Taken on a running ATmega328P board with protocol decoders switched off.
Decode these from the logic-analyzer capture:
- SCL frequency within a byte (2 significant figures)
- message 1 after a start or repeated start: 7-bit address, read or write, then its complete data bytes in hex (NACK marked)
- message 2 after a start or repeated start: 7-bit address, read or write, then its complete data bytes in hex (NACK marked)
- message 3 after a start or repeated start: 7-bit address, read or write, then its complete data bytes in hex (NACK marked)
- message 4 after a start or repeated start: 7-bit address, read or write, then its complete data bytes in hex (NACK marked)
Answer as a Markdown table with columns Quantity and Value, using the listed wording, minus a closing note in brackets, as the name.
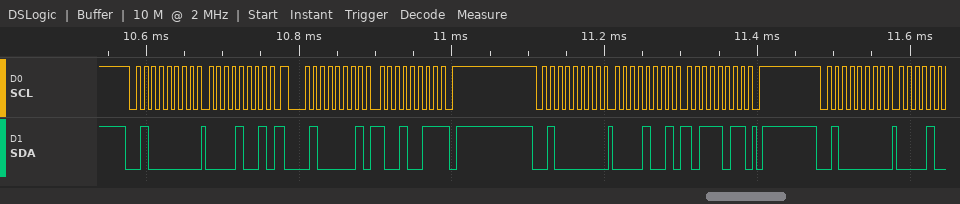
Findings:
| Quantity | Value |
|---|---|
| SCL frequency within a byte | 100 kHz |
| message 1 after a start or repeated start: 7-bit address, read or write, then its complete data bytes in hex | 0x20 write: 09 |
| message 2 after a start or repeated start: 7-bit address, read or write, then its complete data bytes in hex | 0x20 read: 93 NACK |
| message 3 after a start or repeated start: 7-bit address, read or write, then its complete data bytes in hex | 0x20 write: 09 BB |
| message 4 after a start or repeated start: 7-bit address, read or write, then its complete data bytes in hex | 0x20 write |
